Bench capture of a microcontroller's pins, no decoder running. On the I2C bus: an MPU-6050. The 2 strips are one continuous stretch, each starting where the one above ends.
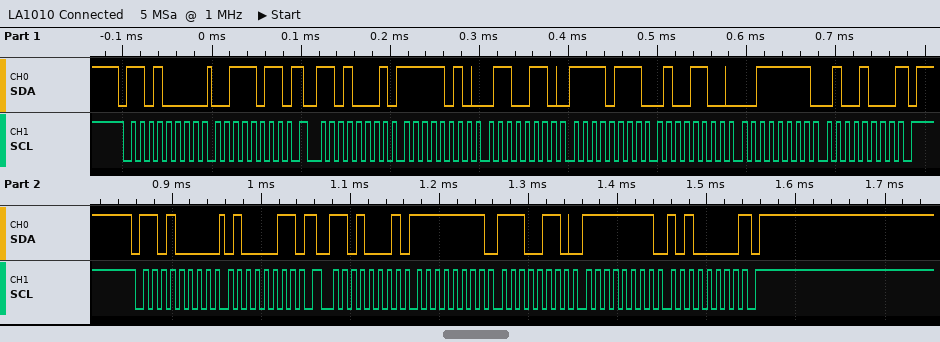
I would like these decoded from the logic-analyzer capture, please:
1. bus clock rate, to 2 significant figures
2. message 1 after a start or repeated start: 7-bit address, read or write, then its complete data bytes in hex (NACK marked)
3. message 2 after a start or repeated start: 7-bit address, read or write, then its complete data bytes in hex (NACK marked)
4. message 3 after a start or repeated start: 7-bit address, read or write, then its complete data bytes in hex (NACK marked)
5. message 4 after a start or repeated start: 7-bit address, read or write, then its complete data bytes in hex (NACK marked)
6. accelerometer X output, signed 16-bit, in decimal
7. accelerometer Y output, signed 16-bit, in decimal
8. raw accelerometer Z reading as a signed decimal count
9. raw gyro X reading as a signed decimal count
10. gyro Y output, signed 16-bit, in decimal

100 kHz
0x68 write: 3B
0x68 read: FA 66 F7 4C 3F 48 NACK
0x68 write: 43
0x68 read: FF E6 FF A0 NACK
-1434
-2228
16200
-26
-96
